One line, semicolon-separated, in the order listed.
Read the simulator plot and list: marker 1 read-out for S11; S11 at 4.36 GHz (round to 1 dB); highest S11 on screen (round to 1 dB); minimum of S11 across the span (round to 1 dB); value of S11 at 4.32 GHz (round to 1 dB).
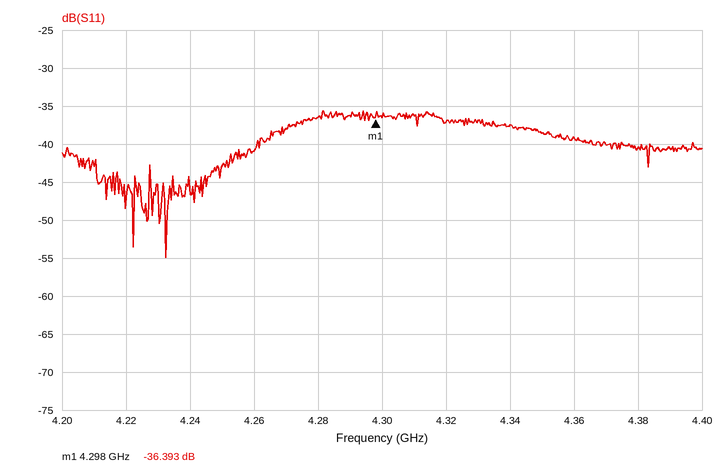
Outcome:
-36.393 dB; -39 dB; -36 dB; -55 dB; -37 dB
